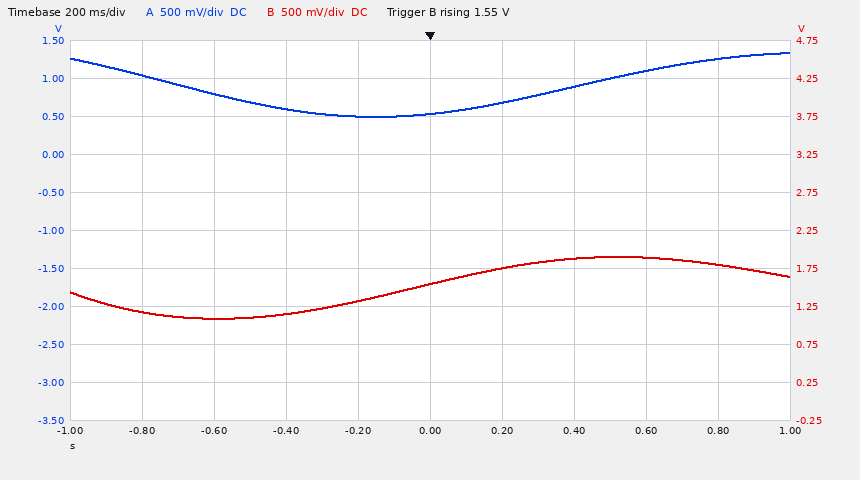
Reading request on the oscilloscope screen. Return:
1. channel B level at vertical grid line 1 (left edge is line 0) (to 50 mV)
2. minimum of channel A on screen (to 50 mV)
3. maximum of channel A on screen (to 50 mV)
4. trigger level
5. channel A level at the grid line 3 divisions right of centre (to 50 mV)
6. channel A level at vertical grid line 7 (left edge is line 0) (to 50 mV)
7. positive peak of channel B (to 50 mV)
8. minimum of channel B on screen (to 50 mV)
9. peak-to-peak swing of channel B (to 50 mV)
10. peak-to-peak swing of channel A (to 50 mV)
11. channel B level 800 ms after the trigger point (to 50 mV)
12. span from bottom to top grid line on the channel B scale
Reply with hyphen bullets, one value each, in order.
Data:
- 1.20 V
- 500 mV
- 1.35 V
- 1.55 V
- 1.10 V
- 900 mV
- 1.90 V
- 1.10 V
- 800 mV
- 850 mV
- 1.80 V
- 5 V
